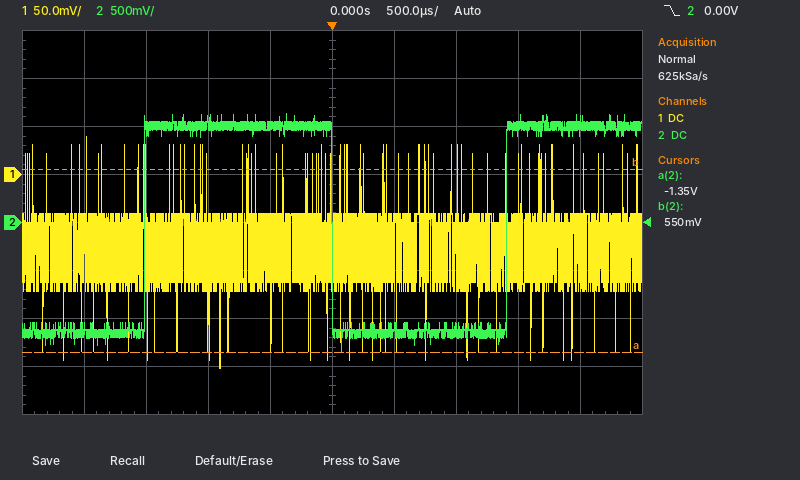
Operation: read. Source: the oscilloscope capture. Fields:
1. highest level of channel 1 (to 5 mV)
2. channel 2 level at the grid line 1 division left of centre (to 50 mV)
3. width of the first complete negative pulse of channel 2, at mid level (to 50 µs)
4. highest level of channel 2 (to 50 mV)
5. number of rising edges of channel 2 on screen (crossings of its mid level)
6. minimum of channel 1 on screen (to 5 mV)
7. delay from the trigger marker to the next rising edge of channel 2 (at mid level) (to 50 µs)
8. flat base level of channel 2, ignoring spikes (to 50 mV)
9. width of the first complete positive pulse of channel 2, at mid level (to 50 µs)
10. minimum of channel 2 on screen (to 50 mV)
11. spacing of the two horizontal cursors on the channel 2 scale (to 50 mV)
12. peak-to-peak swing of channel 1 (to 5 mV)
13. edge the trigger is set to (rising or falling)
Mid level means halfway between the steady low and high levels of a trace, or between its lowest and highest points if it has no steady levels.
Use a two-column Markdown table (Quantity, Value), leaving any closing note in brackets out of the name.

| Quantity | Value |
|---|---|
| highest level of channel 1 | 40 mV |
| channel 2 level at the grid line 1 division left of centre | 1.00 V |
| width of the first complete negative pulse of channel 2, at mid level | 1.40 ms |
| highest level of channel 2 | 1.15 V |
| number of rising edges of channel 2 on screen | 2 |
| minimum of channel 1 on screen | -200 mV |
| delay from the trigger marker to the next rising edge of channel 2 (at mid level) | 1.40 ms |
| flat base level of channel 2, ignoring spikes | -1.15 V |
| width of the first complete positive pulse of channel 2, at mid level | 1.50 ms |
| minimum of channel 2 on screen | -1.35 V |
| spacing of the two horizontal cursors on the channel 2 scale | 1.90 V |
| peak-to-peak swing of channel 1 | 240 mV |
| edge the trigger is set to | falling |
